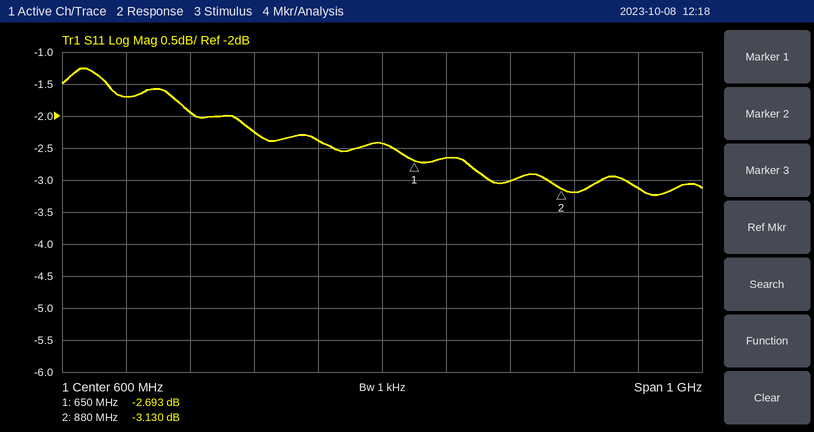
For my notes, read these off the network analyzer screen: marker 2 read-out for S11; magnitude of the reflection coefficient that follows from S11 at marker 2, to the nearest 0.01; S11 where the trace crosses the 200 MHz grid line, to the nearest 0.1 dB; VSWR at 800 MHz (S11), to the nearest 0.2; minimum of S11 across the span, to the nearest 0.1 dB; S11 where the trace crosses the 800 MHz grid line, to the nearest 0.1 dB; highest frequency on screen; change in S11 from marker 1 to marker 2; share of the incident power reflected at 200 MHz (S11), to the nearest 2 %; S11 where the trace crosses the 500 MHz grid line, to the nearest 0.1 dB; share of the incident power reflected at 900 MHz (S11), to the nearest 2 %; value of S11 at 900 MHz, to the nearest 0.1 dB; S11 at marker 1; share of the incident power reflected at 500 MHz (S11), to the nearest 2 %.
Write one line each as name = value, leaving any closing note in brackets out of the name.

marker 2 read-out for S11 = -3.130 dB
magnitude of the reflection coefficient that follows from S11 at marker 2, to the nearest 0.01 = 0.70
S11 where the trace crosses the 200 MHz grid line, to the nearest 0.1 dB = -1.7 dB
VSWR at 800 MHz (S11), to the nearest 0.2 = 5.8
minimum of S11 across the span, to the nearest 0.1 dB = -3.2 dB
S11 where the trace crosses the 800 MHz grid line, to the nearest 0.1 dB = -3.0 dB
highest frequency on screen = 1.1 GHz
change in S11 from marker 1 to marker 2 = -0.437 dB
share of the incident power reflected at 200 MHz (S11), to the nearest 2 % = 68 %
S11 where the trace crosses the 500 MHz grid line, to the nearest 0.1 dB = -2.4 dB
share of the incident power reflected at 900 MHz (S11), to the nearest 2 % = 48 %
value of S11 at 900 MHz, to the nearest 0.1 dB = -3.2 dB
S11 at marker 1 = -2.693 dB
share of the incident power reflected at 500 MHz (S11), to the nearest 2 % = 58 %
